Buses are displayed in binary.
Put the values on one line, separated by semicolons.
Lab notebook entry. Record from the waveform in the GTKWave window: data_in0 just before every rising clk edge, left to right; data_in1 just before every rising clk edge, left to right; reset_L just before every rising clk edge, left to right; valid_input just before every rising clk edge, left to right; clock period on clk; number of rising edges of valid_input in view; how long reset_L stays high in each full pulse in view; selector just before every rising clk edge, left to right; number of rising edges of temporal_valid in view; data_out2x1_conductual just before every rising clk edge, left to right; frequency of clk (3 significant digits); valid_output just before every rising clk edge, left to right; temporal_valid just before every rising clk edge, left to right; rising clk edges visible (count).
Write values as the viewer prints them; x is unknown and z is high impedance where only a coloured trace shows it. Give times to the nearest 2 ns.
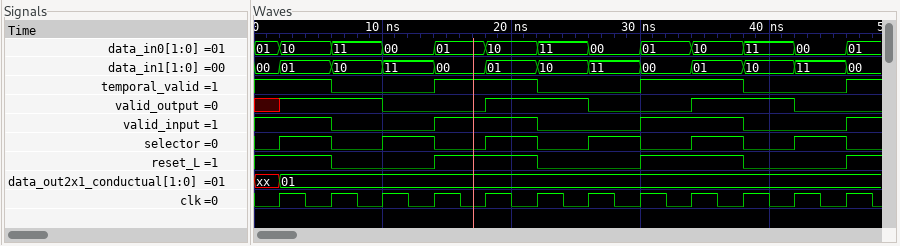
01, 10, 11, 00, 01, 10, 11, 00, 01, 10, 11, 00; 00, 01, 10, 11, 00, 01, 10, 11, 00, 01, 10, 11; 1 1 0 0 1 1 0 0 1 1 0 0; 1 1 0 0 1 1 0 0 1 1 0 0; 4 ns; 3; 8 ns, 8 ns; 0 1 0 1 0 1 0 1 0 1 0 1; 3; xx, 01, 01, 01, 01, 01, 01, 01, 01, 01, 01, 01; 250 MHz; x 1 1 0 0 1 1 0 0 1 1 0; 1 1 0 0 1 1 0 0 1 1 0 0; 12
